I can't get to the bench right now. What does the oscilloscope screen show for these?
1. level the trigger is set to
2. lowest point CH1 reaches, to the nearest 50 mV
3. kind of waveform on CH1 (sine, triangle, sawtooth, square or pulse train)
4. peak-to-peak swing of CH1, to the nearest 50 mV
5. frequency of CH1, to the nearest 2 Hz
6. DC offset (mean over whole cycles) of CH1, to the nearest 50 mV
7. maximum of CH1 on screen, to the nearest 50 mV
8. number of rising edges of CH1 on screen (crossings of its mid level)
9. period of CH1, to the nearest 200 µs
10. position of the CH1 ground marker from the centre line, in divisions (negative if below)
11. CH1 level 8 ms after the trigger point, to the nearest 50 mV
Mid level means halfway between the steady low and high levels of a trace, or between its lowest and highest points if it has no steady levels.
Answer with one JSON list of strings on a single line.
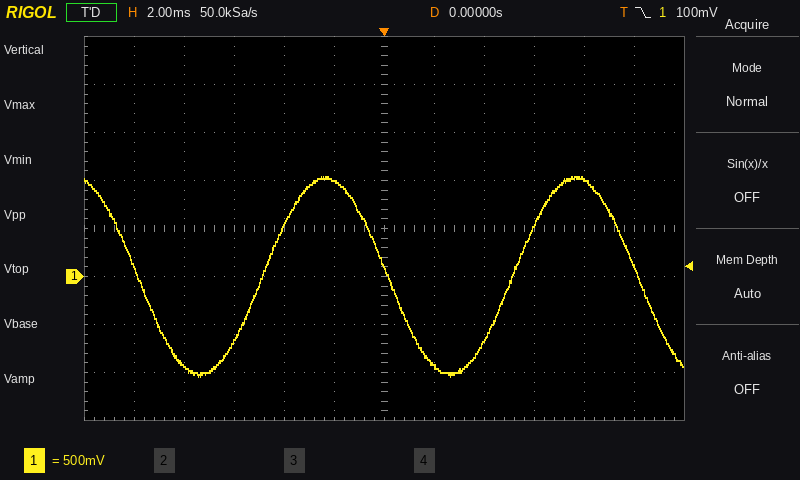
["100 mV", "-1.05 V", "sine", "2.10 V", "100 Hz", "0 mV", "1.05 V", "2", "10.0 ms", "-1.0 div", "1.00 V"]
